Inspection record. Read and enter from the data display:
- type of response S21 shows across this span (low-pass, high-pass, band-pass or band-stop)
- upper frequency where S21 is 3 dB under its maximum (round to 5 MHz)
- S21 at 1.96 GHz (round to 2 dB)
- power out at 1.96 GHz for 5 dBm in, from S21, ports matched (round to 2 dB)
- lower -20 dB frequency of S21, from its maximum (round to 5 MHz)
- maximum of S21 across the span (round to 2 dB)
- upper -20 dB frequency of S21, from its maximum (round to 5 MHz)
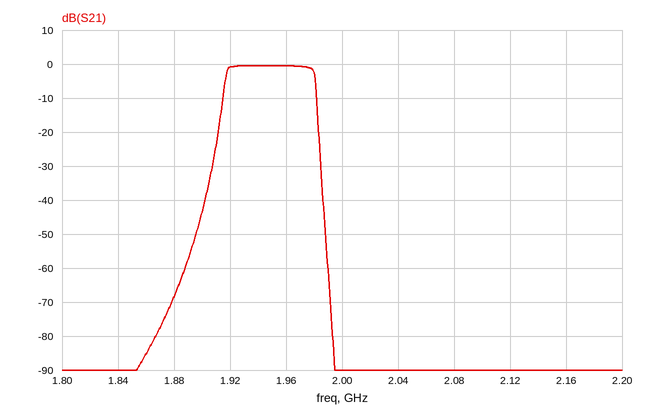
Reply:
band-pass
1.980 GHz
0 dB
4 dBm
1.910 GHz
0 dB
1.985 GHz
